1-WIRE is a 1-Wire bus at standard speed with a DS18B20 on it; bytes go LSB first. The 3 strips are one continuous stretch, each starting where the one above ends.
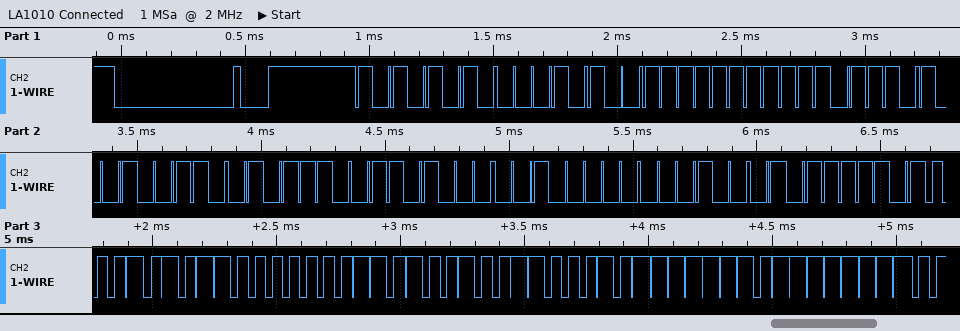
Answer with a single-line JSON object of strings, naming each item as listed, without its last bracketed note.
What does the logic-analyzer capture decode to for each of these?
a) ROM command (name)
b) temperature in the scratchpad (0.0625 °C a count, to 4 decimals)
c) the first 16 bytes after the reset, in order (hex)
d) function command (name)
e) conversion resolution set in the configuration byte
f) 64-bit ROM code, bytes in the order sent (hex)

{"ROM command": "Match ROM", "temperature in the scratchpad": "26.5000 °C", "the first 16 bytes after the reset, in order": "55 28 FF 77 C9 74 16 04 88 BE A8 01 4B 46 7F FF", "function command": "Read Scratchpad", "conversion resolution set in the configuration byte": "12 bits", "64-bit ROM code, bytes in the order sent": "28 FF 77 C9 74 16 04 88"}
